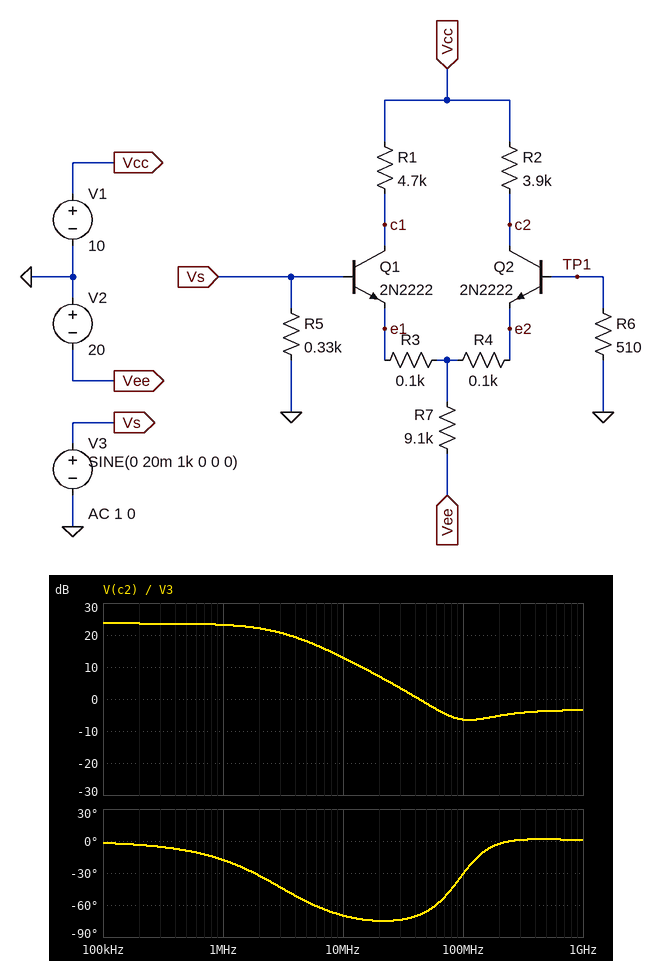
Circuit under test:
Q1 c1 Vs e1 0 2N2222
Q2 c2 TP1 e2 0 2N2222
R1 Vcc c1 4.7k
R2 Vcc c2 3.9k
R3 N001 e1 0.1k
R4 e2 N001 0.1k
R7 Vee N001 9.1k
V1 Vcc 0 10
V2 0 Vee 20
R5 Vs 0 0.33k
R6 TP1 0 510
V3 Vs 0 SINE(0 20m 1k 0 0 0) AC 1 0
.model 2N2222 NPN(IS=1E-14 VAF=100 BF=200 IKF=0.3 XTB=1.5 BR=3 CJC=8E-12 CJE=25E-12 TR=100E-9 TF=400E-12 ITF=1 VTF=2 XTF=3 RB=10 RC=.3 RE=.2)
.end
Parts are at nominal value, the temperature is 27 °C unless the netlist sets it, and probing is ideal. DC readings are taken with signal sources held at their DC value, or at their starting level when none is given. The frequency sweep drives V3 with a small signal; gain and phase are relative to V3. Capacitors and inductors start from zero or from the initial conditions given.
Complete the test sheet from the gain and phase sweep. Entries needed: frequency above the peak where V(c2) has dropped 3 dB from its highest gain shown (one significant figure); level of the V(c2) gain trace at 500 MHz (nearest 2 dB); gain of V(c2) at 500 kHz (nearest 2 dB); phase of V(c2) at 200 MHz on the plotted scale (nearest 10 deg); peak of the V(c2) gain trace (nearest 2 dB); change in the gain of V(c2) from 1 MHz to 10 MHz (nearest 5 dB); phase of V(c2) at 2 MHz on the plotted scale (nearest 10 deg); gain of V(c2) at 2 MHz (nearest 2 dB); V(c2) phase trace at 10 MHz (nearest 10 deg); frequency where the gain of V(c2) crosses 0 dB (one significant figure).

3 MHz
-4 dB
24 dB
0 deg
24 dB
-10 dB
-30 deg
22 dB
-70 deg
40 MHz
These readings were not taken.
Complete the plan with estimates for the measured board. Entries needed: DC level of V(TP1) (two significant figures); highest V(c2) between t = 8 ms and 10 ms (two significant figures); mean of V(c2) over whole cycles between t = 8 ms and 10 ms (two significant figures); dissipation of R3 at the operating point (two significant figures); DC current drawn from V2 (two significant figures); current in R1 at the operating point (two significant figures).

-2.5 mV
6.2 V
5.9 V
110 µW
2.1 mA
1.1 mA
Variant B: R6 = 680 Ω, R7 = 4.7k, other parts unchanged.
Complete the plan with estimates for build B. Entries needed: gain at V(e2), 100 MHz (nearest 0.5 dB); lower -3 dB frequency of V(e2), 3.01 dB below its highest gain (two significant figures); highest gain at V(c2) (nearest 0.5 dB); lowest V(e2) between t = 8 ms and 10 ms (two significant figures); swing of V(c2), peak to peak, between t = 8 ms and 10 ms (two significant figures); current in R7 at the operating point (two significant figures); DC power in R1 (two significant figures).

-3.0 dB
1.8 MHz
24.5 dB
-680 mV
660 mV
4.1 mA
20 mW
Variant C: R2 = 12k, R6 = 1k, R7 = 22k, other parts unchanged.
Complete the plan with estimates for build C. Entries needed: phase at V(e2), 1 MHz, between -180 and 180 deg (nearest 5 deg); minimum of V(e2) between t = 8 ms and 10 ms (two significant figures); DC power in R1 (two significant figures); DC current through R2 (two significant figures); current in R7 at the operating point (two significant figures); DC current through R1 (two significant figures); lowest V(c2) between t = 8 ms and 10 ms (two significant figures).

25 deg
-640 mV
930 µW
430 µA
880 µA
450 µA
4.1 V
